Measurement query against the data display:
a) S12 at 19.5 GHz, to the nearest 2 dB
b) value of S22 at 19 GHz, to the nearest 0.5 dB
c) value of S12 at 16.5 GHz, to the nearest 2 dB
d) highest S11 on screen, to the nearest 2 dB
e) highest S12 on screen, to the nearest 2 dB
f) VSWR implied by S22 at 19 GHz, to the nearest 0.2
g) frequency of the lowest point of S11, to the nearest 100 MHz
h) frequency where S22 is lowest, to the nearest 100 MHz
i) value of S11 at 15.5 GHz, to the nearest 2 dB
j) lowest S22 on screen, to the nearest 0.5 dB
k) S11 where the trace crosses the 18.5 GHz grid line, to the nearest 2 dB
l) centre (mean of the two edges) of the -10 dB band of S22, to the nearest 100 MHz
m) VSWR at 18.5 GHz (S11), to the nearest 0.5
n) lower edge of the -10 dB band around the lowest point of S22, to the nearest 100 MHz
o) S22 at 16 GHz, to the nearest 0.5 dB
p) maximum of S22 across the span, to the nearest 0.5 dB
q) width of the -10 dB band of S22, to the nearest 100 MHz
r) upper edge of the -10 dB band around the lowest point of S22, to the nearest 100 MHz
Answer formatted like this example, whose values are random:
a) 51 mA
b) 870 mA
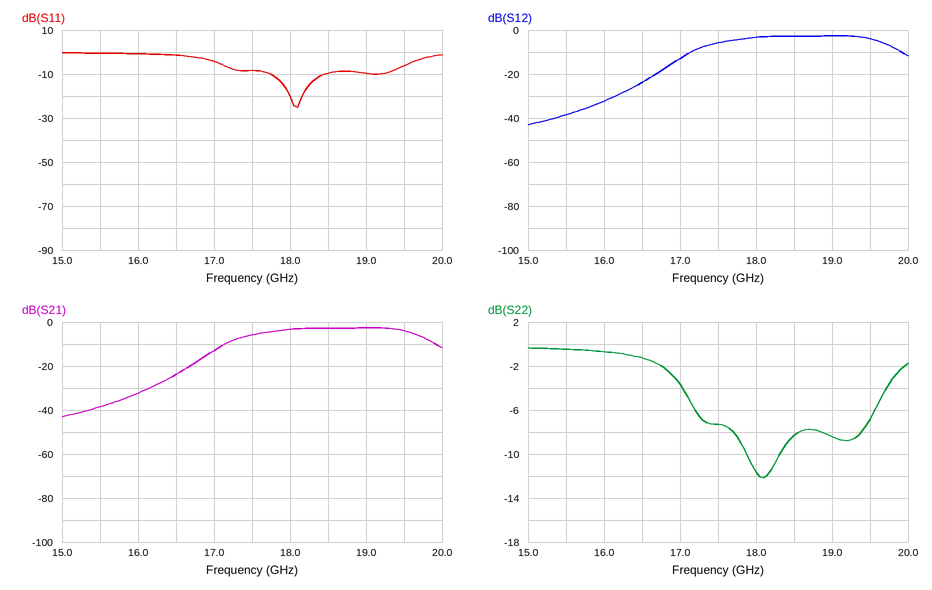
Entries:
a) -4 dB
b) -8.5 dB
c) -24 dB
d) 0 dB
e) -2 dB
f) 2.2
g) 18.1 GHz
h) 18.1 GHz
i) 0 dB
j) -12.0 dB
k) -10 dB
l) 18.1 GHz
m) 2.0
n) 17.9 GHz
o) -0.5 dB
p) -0.5 dB
q) 400 MHz
r) 18.3 GHz
